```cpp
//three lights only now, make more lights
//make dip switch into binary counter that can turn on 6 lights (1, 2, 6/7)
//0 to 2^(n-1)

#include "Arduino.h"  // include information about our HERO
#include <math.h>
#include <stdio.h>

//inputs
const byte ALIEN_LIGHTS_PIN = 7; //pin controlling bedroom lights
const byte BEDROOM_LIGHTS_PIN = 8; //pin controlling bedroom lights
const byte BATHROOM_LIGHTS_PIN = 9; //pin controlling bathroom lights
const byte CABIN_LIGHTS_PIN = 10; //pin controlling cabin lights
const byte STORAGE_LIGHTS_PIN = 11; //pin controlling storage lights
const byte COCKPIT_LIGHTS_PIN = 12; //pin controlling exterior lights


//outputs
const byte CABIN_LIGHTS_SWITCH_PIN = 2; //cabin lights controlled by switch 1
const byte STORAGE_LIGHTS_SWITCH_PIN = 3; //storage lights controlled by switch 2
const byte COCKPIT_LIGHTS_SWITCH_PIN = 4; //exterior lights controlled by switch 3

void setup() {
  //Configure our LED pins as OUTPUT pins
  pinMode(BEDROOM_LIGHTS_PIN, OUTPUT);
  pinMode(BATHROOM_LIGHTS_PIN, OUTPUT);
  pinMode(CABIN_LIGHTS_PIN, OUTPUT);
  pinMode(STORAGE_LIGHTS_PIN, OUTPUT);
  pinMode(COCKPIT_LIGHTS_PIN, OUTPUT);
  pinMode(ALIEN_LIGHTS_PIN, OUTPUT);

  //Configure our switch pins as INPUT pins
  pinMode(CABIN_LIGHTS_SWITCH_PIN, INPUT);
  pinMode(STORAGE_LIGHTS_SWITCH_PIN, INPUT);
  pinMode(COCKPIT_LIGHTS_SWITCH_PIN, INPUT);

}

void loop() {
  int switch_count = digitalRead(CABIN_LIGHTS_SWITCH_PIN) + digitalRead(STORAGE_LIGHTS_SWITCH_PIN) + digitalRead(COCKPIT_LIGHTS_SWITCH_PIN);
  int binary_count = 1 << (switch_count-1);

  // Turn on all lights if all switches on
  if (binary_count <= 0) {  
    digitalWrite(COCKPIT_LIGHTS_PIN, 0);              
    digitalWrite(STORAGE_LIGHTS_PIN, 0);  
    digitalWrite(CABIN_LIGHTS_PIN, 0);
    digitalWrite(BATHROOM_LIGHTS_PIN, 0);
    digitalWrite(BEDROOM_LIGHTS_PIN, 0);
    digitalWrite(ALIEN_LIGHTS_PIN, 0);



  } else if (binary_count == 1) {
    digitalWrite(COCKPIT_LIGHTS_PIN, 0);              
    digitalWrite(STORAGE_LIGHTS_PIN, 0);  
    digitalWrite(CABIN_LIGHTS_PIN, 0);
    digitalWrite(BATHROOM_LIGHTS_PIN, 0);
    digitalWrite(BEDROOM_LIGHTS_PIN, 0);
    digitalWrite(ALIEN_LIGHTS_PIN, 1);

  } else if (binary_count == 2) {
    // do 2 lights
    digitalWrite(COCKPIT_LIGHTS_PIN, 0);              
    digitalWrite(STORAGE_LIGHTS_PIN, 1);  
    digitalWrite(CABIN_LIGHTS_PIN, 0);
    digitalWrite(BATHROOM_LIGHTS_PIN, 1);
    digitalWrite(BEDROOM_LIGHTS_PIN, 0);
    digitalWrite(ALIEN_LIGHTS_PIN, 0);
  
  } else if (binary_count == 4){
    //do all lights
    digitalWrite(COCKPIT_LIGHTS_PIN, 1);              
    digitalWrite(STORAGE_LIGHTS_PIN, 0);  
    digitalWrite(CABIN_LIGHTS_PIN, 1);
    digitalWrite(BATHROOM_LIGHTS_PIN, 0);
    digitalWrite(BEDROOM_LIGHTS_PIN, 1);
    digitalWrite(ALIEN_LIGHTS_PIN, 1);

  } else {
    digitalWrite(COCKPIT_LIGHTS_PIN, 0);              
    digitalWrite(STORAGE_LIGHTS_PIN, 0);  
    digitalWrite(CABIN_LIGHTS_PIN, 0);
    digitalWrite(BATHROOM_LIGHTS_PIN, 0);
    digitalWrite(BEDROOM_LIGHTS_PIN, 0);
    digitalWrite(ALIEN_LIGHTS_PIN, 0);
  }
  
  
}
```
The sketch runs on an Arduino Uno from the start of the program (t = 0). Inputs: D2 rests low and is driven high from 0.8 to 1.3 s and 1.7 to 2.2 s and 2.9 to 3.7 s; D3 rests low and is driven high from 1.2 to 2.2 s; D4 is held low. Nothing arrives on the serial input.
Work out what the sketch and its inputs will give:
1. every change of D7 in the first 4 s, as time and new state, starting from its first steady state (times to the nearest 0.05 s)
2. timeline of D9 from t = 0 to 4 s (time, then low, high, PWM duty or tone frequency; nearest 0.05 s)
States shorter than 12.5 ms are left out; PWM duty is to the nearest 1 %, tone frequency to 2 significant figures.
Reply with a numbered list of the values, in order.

1. 0 s low; 0.8 s high; 1.2 s low; 1.3 s high; 1.7 s low; 2.9 s high; 3.7 s low
2. 0 s low; 1.2 s high; 1.3 s low; 1.7 s high; 2.2 s low
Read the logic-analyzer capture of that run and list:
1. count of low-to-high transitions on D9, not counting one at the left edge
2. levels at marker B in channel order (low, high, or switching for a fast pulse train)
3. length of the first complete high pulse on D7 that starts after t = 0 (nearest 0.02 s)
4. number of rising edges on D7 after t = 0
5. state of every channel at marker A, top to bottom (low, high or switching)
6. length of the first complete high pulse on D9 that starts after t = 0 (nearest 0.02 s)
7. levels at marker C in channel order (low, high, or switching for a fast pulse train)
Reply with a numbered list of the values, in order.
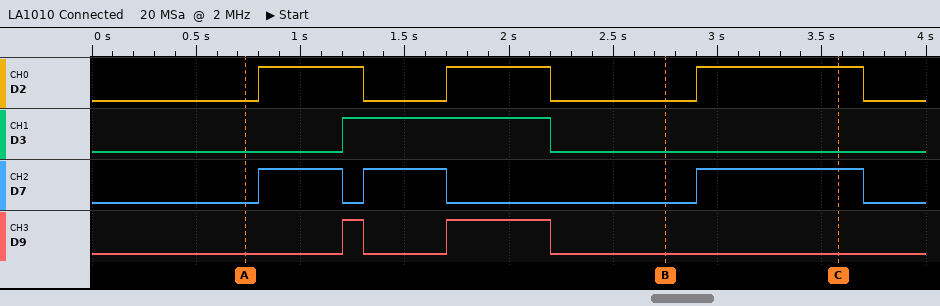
1. 2
2. D2 low, D3 low, D7 low, D9 low
3. 0.40 s
4. 3
5. D2 low, D3 low, D7 low, D9 low
6. 0.10 s
7. D2 high, D3 low, D7 high, D9 low
